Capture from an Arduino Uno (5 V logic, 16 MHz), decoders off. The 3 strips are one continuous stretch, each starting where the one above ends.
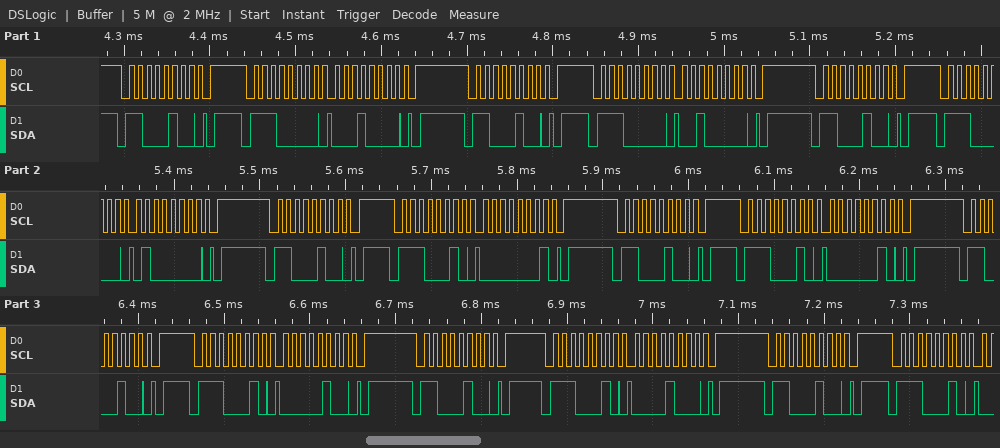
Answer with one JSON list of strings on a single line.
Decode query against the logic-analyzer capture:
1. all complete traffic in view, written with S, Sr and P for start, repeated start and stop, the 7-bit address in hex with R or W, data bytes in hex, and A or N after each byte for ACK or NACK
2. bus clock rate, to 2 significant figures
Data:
["S 62W A P S 70W A 10 A P S 62W A P S 70W A 20 A P S 62W A P S 70W A 40 A P S 62W A P S 71W A 01 A P S 62W A P S 71W A 02 A P S 62W A P S 71W A 04 A P S 62W A P S 71W A 08 A P S 62W A P S 71W A", "100 kHz"]
